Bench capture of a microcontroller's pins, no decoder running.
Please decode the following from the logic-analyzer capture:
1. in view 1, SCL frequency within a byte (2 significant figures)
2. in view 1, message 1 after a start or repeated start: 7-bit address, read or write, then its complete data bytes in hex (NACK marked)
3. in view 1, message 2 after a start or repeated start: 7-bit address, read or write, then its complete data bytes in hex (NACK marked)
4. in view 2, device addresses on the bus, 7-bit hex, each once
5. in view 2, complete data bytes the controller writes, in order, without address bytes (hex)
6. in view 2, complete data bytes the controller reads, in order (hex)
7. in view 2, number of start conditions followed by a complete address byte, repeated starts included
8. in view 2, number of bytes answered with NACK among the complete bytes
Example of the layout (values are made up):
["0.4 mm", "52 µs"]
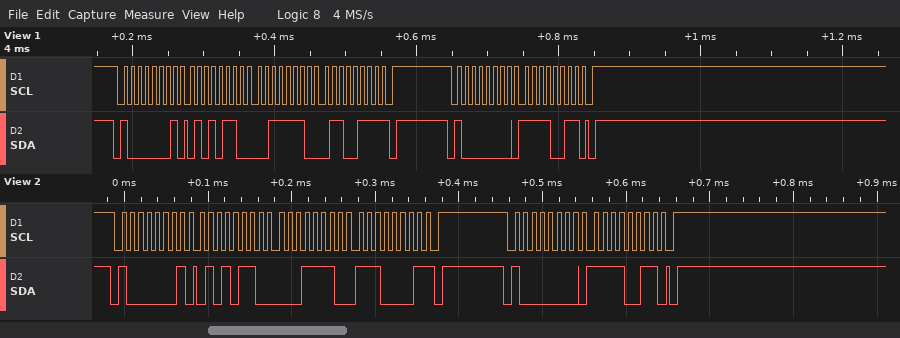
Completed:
["100 kHz", "0x40 read: 56 3E 67 NACK", "0x40 write: F3", "0x40", "F3", "56 1E E1", "2", "1"]
